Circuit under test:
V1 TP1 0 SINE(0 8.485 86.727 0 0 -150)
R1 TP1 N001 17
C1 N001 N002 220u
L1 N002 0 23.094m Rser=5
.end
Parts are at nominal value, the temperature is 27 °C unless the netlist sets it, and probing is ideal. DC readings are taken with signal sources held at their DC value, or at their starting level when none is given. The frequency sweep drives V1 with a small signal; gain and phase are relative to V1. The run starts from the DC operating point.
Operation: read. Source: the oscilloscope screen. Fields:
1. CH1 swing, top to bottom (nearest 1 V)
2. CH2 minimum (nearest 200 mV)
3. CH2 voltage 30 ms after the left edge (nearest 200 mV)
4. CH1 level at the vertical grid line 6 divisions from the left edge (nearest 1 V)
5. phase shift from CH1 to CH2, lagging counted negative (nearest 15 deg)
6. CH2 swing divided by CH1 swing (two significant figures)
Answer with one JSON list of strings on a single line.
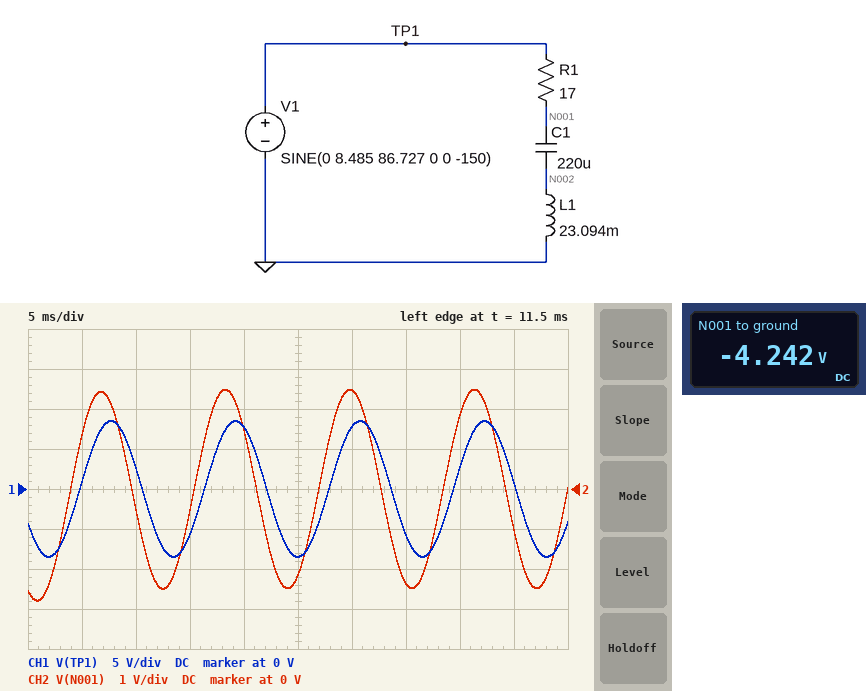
["17 V", "-2.8 V", "2.4 V", "8 V", "30 deg", "0.31"]
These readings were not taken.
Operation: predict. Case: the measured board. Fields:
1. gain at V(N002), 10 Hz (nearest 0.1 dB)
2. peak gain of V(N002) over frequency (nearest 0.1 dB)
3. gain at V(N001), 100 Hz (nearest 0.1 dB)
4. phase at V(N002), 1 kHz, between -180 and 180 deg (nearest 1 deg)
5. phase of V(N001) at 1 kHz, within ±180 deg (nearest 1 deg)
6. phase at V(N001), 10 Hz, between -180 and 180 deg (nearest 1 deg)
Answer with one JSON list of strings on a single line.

["-23.1 dB", "0 dB", "-8.4 dB", "7 deg", "7 deg", "-13 deg"]
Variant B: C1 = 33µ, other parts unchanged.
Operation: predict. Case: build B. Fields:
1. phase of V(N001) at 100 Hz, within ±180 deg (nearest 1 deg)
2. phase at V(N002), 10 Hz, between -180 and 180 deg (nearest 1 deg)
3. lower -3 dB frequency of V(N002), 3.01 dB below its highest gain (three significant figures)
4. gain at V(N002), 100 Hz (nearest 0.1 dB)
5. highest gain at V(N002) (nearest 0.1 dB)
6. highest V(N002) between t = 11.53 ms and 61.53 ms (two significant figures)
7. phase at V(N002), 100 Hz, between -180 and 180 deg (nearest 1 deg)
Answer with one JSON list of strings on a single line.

["-25 deg", "104 deg", "152 Hz", "-8.4 dB", "2.5 dB", "2.4 V", "128 deg"]
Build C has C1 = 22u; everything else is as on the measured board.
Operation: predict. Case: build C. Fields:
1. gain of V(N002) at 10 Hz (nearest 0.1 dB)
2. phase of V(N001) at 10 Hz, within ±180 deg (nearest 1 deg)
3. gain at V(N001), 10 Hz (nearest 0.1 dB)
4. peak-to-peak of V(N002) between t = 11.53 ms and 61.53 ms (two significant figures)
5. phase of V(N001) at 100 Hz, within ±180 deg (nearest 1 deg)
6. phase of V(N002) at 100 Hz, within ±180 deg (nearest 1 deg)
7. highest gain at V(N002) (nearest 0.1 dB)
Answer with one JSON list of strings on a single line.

["-42.8 dB", "-1 deg", "0 dB", "3.1 V", "-16 deg", "140 deg", "4.0 dB"]
